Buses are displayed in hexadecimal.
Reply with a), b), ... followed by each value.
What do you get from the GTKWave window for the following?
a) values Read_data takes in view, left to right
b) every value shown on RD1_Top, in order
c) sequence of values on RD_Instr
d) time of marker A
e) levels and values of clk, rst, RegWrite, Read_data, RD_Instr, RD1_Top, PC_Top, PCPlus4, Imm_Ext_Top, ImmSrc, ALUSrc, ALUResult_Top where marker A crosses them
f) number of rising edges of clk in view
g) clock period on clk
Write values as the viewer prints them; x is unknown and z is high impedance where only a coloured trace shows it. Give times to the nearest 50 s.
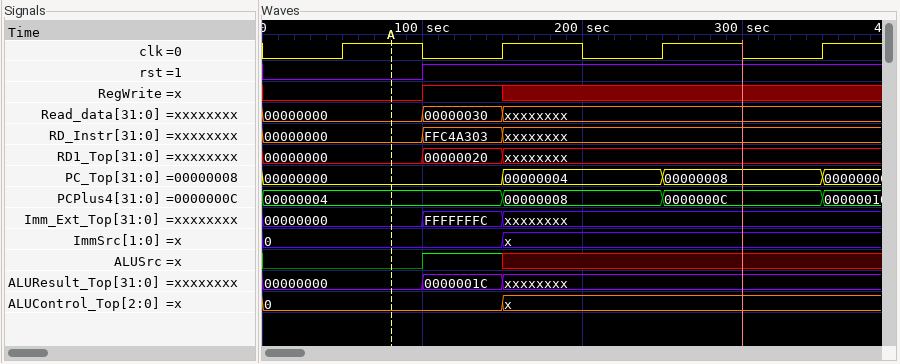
a) 00000000, 00000030, xxxxxxxx
b) 00000000, 00000020, xxxxxxxx
c) 00000000, FFC4A303, xxxxxxxx
d) 100 s
e) clk=1, rst=0, RegWrite=0, Read_data=00000000, RD_Instr=00000000, RD1_Top=00000000, PC_Top=00000000, PCPlus4=00000004, Imm_Ext_Top=00000000, ImmSrc=0, ALUSrc=0, ALUResult_Top=00000000
f) 4
g) 100 s
